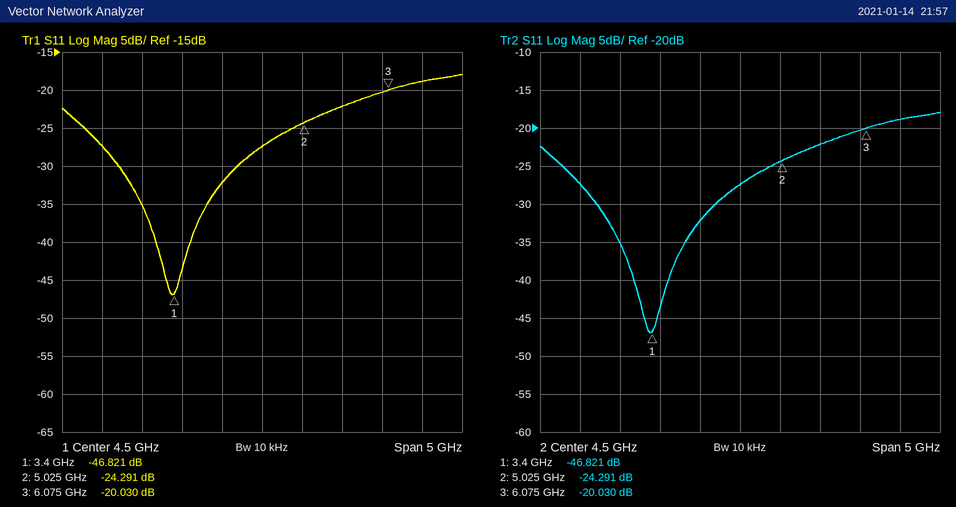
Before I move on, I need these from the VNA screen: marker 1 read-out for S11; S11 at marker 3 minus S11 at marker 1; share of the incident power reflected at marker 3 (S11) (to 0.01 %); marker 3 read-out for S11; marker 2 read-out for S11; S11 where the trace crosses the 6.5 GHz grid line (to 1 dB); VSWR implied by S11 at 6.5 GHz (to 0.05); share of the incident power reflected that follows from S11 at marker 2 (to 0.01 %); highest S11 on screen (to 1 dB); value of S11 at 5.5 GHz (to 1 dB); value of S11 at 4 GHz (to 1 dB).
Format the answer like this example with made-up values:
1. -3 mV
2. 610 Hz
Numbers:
1. -46.821 dB
2. 26.791 dB
3. 0.99 %
4. -20.030 dB
5. -24.291 dB
6. -19 dB
7. 1.25
8. 0.37 %
9. -18 dB
10. -22 dB
11. -32 dB
